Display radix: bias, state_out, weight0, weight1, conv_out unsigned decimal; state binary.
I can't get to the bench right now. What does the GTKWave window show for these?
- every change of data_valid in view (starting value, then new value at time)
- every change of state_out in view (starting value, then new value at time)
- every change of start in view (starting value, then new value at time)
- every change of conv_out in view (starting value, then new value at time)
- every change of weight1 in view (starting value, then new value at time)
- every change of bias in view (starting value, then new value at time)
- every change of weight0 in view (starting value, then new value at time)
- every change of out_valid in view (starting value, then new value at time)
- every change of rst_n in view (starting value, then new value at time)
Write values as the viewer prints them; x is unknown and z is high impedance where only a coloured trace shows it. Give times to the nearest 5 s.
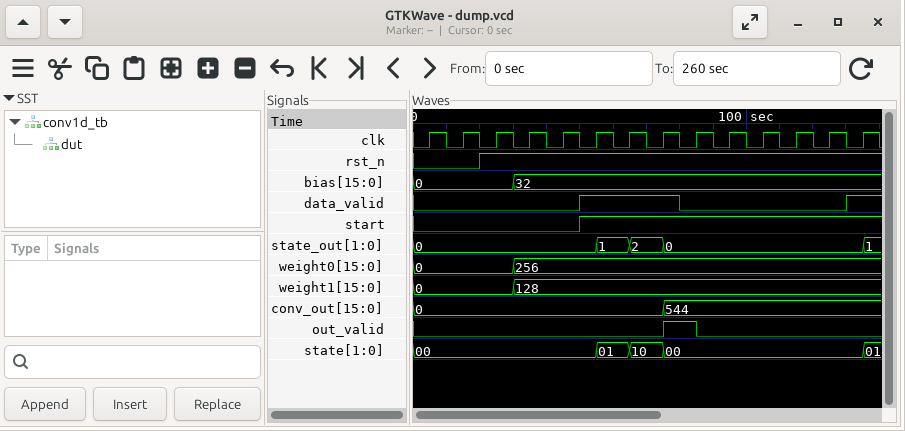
0, 1 at 50 s, 0 at 80 s, 1 at 130 s
0, 1 at 55 s, 2 at 65 s, 0 at 75 s, 1 at 135 s
0, 1 at 50 s
0, 544 at 75 s
0, 128 at 30 s
0, 32 at 30 s
0, 256 at 30 s
0, 1 at 75 s, 0 at 85 s
0, 1 at 20 s
